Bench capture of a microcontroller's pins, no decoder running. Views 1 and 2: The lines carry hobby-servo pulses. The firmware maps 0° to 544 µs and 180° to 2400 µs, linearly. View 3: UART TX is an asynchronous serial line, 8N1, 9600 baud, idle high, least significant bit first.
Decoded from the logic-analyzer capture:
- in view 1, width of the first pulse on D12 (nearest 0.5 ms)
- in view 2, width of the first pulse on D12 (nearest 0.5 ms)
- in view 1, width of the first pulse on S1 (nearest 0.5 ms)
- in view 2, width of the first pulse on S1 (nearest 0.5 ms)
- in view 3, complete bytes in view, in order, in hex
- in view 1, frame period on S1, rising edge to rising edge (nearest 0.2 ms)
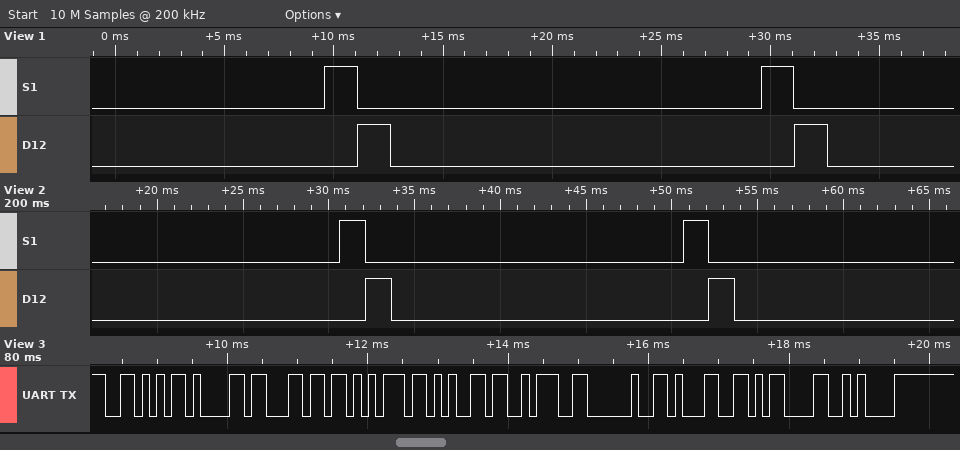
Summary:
1.5 ms
1.5 ms
1.5 ms
1.5 ms
0x56 0x61 0x6C 0x75 0x65 0x3A 0x20 0x31 0x0D 0x0A
20.0 ms
